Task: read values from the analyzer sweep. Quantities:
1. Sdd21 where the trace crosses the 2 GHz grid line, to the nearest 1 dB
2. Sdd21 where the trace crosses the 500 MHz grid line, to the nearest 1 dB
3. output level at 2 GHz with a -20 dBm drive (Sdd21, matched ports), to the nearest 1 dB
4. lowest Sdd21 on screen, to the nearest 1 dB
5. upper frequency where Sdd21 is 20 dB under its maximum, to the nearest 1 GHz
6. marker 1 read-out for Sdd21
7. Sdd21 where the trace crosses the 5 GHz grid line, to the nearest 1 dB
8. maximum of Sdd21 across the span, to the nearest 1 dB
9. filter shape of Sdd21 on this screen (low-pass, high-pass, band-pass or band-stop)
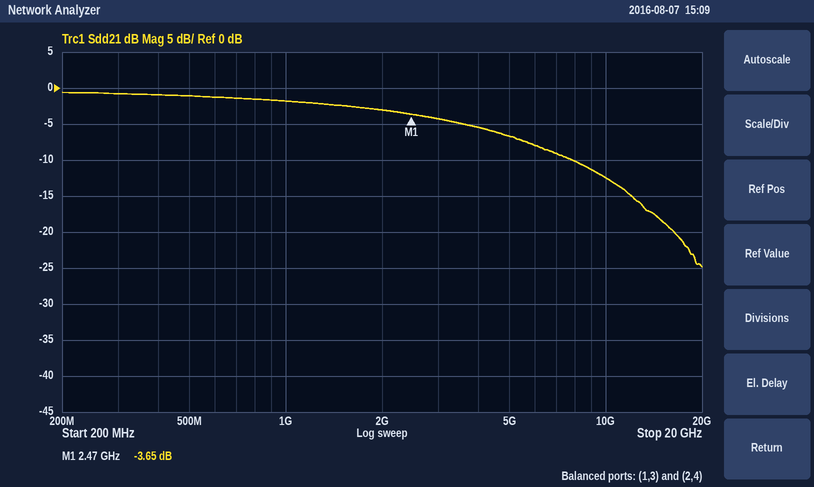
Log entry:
-3 dB
-1 dB
-23 dBm
-25 dB
17 GHz
-3.65 dB
-7 dB
-1 dB
low-pass
